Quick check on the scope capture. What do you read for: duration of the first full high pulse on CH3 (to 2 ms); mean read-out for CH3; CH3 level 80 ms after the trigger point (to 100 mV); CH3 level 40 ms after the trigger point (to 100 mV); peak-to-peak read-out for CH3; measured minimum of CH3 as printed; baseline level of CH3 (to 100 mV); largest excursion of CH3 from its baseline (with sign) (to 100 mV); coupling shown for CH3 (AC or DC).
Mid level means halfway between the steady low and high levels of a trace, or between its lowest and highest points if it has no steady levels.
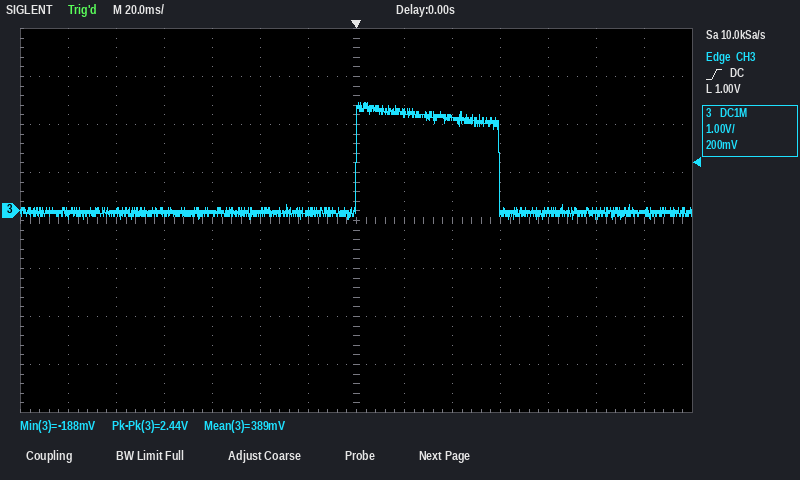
60 ms
389 mV
0.0 V
1.9 V
2.44 V
-188 mV
0.0 V
+2.3 V
DC
